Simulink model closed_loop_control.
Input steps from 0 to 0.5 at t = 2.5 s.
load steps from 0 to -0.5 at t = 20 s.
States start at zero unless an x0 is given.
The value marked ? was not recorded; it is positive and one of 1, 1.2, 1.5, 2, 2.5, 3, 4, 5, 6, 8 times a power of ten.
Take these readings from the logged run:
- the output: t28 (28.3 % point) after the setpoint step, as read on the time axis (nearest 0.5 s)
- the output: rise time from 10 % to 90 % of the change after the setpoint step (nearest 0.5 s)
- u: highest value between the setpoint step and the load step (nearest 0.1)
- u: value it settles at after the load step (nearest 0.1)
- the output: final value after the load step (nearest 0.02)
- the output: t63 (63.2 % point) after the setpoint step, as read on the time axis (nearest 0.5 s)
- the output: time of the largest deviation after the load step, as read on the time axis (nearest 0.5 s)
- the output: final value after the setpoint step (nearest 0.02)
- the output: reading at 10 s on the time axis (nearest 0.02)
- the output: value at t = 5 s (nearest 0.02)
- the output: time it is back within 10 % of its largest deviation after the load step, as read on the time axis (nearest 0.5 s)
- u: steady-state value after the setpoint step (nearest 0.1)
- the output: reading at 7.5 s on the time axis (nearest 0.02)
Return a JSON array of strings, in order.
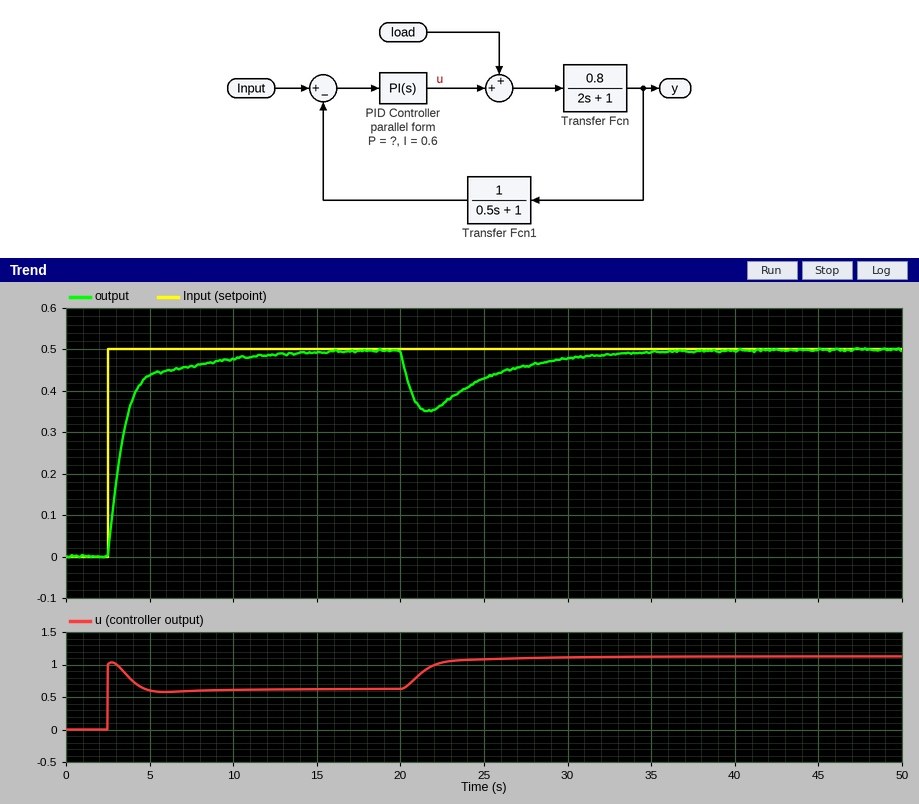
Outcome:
["3.0 s", "3.5 s", "1.0", "1.1", "0.50", "3.5 s", "21.5 s", "0.50", "0.48", "0.44", "32.0 s", "0.6", "0.46"]
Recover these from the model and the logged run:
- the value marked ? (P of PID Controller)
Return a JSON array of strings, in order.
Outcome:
["2"]
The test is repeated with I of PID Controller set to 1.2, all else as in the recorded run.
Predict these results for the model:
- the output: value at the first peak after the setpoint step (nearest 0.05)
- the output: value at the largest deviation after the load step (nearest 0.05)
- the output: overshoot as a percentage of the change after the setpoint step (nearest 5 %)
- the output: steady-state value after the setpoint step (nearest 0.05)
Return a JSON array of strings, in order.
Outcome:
["0.55", "0.35", "10 %", "0.50"]
